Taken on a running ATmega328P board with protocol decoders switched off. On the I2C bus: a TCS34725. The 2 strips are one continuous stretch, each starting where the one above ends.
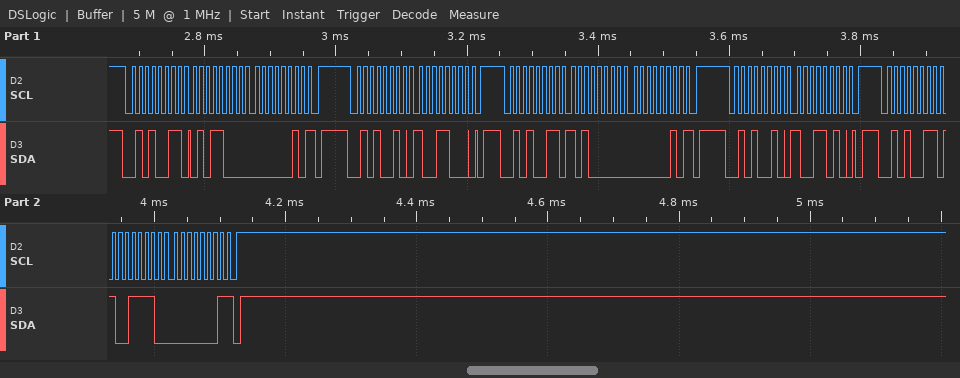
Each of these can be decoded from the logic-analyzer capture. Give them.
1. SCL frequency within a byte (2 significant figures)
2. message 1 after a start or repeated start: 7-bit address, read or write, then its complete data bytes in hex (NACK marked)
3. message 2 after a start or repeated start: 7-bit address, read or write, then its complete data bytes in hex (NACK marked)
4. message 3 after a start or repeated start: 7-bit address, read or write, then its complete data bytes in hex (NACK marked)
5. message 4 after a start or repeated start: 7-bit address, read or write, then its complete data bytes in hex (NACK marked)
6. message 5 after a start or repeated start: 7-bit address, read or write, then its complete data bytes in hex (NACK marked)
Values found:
100 kHz
0x29 read: 58 02 NACK
0x29 write: 98
0x29 read: A0 02 NACK
0x29 write: 9A
0x29 read: 9E 01 NACK
